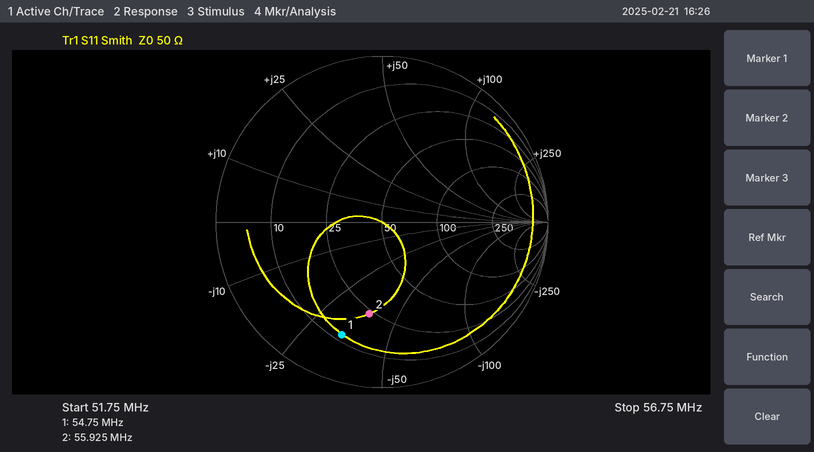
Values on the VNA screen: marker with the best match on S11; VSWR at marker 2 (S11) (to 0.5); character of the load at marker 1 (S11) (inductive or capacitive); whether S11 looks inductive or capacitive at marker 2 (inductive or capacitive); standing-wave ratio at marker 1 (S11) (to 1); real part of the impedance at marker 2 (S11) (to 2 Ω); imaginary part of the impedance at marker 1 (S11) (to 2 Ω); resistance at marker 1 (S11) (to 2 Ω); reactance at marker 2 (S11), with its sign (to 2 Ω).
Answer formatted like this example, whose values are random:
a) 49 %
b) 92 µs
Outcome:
a) marker 2
b) 3.5
c) capacitive
d) capacitive
e) 6
f) 24 Ω
g) -34 Ω
h) 12 Ω
i) -38 Ω
